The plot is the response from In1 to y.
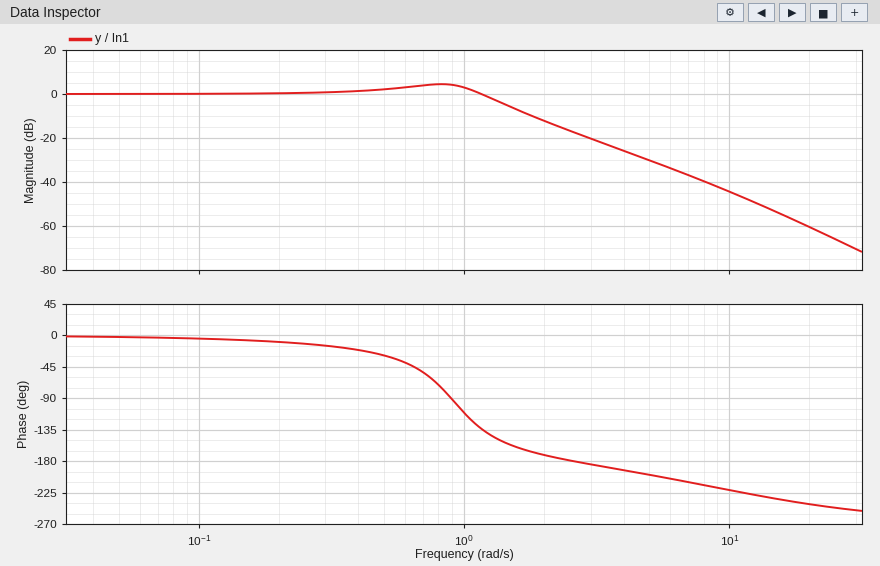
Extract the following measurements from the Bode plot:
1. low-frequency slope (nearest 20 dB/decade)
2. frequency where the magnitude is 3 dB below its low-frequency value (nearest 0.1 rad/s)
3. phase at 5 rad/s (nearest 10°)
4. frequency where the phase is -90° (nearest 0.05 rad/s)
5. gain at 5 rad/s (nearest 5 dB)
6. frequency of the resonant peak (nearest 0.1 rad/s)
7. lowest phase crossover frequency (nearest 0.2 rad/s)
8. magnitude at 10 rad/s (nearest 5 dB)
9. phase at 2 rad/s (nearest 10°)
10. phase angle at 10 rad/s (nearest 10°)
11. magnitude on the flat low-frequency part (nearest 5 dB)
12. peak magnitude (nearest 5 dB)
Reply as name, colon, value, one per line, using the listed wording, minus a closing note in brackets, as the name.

low-frequency slope: 0 dB/decade
frequency where the magnitude is 3 dB below its low-frequency value: 1.3 rad/s
phase at 5 rad/s: -200°
frequency where the phase is -90°: 0.90 rad/s
gain at 5 rad/s: -30 dB
frequency of the resonant peak: 0.8 rad/s
lowest phase crossover frequency: 2.6 rad/s
magnitude at 10 rad/s: -45 dB
phase at 2 rad/s: -170°
phase angle at 10 rad/s: -220°
magnitude on the flat low-frequency part: 0 dB
peak magnitude: 5 dB
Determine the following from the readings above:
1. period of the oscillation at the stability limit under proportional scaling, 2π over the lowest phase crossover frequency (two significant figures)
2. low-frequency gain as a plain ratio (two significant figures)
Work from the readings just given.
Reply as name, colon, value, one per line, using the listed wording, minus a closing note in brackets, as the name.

period of the oscillation at the stability limit under proportional scaling, 2π over the lowest phase crossover frequency: 2.4 s
low-frequency gain as a plain ratio: 1.0
